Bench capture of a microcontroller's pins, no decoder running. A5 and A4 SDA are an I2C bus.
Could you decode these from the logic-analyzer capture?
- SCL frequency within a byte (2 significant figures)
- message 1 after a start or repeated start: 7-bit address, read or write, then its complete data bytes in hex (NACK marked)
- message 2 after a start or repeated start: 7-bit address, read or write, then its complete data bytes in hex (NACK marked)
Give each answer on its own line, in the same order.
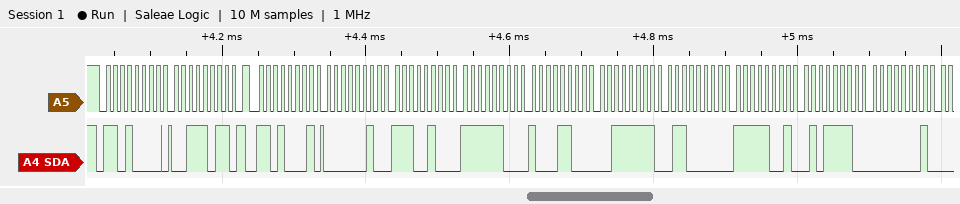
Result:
100 kHz
0x68 write: 3B
0x68 read: 02 E4 FC 8C 3F 60 F9 5E 01
